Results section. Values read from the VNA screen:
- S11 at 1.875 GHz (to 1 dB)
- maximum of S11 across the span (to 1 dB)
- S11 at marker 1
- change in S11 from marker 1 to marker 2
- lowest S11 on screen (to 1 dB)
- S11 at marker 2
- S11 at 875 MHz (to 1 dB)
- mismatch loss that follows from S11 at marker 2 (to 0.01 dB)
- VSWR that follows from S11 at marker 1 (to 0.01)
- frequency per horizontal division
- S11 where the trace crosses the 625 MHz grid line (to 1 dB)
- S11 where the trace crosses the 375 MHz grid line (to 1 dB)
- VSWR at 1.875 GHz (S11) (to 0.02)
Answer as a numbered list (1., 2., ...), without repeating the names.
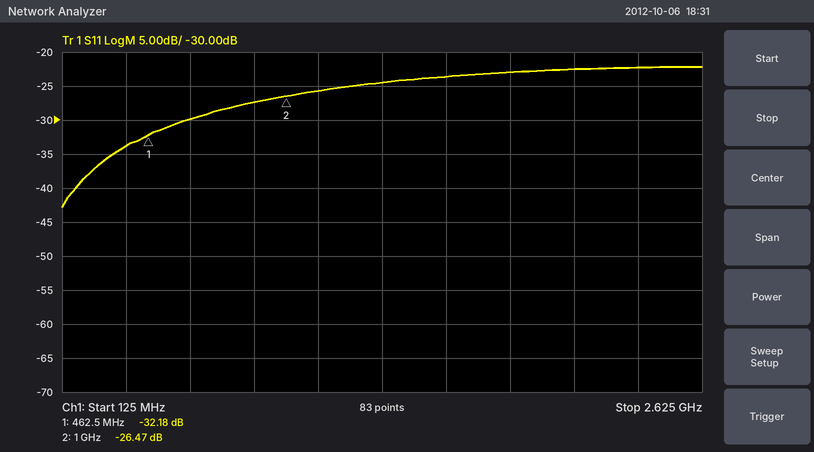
1. -23 dB
2. -22 dB
3. -32.18 dB
4. 5.71 dB
5. -43 dB
6. -26.47 dB
7. -27 dB
8. 0.01 dB
9. 1.05
10. 250 MHz
11. -30 dB
12. -34 dB
13. 1.16
